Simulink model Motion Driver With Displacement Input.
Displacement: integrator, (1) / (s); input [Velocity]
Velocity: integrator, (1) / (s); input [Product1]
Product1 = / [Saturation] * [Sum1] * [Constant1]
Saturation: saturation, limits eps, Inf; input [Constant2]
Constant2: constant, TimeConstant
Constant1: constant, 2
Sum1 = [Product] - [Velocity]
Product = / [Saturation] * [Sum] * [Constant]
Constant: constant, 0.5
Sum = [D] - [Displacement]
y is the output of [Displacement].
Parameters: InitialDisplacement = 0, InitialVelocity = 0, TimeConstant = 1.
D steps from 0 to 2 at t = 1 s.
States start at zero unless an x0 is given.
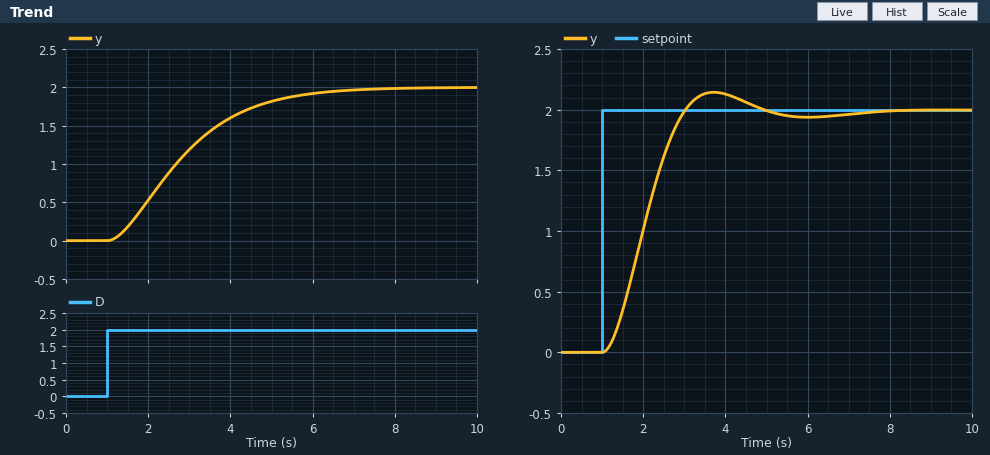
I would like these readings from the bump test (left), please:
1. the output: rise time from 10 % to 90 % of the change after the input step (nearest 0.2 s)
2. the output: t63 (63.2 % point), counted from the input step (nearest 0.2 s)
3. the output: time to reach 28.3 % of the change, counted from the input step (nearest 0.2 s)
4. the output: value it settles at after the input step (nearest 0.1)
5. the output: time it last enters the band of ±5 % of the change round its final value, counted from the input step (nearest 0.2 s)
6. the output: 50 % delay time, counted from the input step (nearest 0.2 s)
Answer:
3.4 s
2.2 s
1.0 s
2.0
4.8 s
1.6 s
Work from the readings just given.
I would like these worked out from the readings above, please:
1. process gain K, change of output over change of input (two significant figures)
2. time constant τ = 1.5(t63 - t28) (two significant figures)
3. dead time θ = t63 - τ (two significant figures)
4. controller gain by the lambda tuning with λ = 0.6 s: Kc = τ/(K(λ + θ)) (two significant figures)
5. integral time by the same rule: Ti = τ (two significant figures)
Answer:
1.0
1.8 s
0.40 s
1.8
1.8 s
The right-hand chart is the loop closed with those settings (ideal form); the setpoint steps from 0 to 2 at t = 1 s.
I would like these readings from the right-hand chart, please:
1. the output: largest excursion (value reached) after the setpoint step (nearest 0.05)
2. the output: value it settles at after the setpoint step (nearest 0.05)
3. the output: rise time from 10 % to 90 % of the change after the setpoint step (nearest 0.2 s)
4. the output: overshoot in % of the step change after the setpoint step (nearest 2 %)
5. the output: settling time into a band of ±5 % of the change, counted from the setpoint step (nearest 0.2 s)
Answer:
2.15
2.00
1.4 s
8 %
3.2 s
